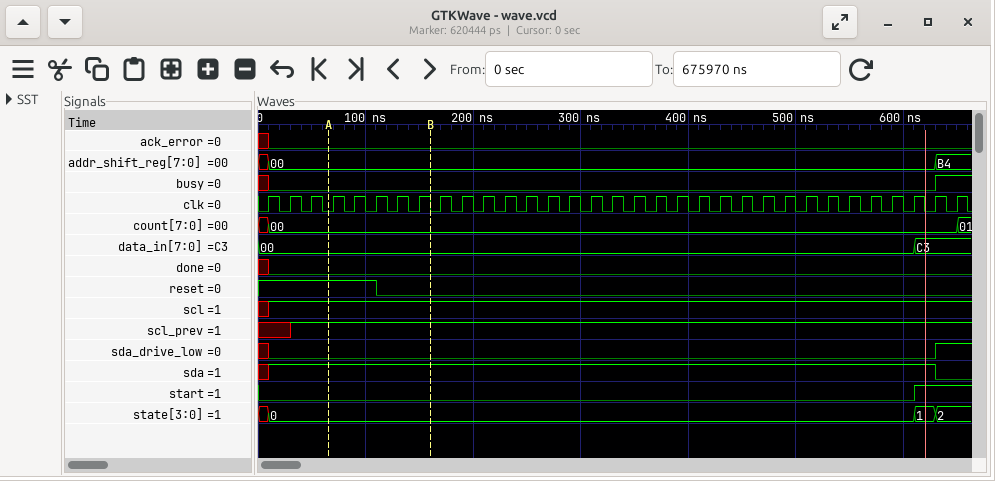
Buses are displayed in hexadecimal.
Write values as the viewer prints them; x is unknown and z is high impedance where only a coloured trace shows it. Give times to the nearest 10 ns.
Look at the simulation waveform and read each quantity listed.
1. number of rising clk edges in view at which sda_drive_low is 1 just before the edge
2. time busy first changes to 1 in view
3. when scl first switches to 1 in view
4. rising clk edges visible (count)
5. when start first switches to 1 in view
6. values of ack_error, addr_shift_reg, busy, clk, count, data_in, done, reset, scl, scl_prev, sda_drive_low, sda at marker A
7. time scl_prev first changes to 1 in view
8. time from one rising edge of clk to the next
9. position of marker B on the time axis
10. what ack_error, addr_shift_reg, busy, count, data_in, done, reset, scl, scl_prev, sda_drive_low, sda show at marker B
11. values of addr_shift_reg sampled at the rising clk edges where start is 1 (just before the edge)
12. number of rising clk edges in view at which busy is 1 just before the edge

1
630 ns
10 ns
33
610 ns
ack_error=0, addr_shift_reg=00, busy=0, clk=0, count=00, data_in=00, done=0, reset=1, scl=1, scl_prev=1, sda_drive_low=0, sda=1
30 ns
20 ns
160 ns
ack_error=0, addr_shift_reg=00, busy=0, count=00, data_in=00, done=0, reset=0, scl=1, scl_prev=1, sda_drive_low=0, sda=1
00, B4
1
